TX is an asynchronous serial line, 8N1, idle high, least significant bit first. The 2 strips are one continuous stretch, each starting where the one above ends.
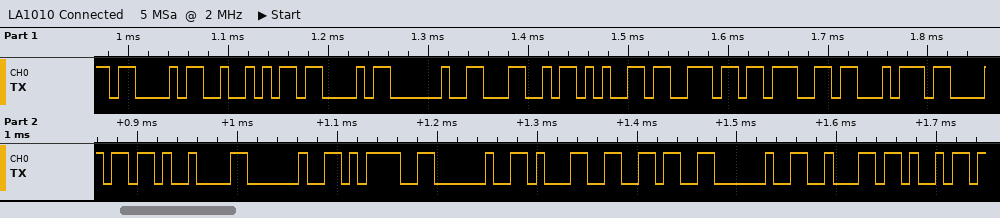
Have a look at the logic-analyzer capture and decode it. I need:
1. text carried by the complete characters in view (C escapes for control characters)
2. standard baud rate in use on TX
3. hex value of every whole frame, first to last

"CRC Length\t = 16 bi"
115200 baud
43 52 43 20 4C 65 6E 67 74 68 09 20 3D 20 31 36 20 62 69
